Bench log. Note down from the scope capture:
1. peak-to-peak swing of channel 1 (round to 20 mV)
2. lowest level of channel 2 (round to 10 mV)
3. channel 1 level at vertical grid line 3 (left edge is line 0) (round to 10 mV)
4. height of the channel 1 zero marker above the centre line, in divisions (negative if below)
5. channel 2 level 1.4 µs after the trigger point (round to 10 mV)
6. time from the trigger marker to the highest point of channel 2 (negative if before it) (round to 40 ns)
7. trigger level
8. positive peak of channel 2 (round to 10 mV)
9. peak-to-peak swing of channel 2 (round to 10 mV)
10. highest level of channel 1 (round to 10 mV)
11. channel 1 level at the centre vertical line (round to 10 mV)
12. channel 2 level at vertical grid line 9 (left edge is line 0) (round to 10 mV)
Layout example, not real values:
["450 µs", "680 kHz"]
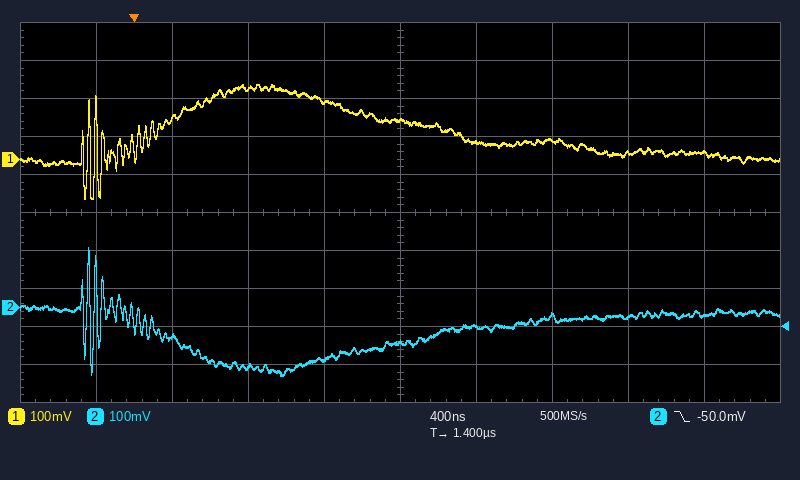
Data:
["300 mV", "-180 mV", "190 mV", "+1.4 div", "-90 mV", "-240 ns", "-50.0 mV", "160 mV", "340 mV", "200 mV", "100 mV", "-20 mV"]
